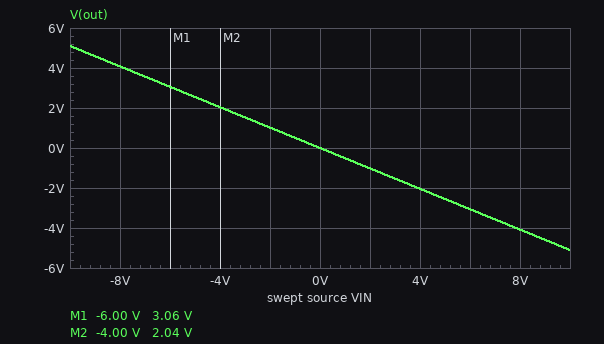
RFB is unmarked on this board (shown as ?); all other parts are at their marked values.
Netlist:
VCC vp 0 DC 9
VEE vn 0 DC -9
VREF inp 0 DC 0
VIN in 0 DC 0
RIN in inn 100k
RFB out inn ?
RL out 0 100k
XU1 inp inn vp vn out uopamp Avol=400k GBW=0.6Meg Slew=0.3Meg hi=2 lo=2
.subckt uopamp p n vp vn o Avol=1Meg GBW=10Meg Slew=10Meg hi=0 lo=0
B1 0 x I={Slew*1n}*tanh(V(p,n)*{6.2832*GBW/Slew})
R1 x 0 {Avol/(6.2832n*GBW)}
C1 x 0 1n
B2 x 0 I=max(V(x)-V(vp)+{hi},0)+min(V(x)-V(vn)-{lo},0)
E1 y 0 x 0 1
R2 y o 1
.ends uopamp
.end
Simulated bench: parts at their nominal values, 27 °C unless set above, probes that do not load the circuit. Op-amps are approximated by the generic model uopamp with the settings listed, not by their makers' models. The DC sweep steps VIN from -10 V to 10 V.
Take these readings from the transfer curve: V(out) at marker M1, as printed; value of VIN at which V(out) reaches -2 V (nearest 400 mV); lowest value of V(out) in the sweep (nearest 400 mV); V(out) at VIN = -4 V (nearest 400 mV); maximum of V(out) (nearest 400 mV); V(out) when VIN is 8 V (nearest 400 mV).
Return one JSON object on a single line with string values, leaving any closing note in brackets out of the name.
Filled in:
{"V(out) at marker M1, as printed": "3.06 V", "value of VIN at which V(out) reaches -2 V": "4.0 V", "lowest value of V(out) in the sweep": "-5.2 V", "V(out) at VIN = -4 V": "2.0 V", "maximum of V(out)": "5.2 V", "V(out) when VIN is 8 V": "-4.0 V"}
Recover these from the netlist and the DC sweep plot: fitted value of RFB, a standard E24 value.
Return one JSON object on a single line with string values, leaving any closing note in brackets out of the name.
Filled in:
{"fitted value of RFB, a standard E24 value": "51 kΩ"}
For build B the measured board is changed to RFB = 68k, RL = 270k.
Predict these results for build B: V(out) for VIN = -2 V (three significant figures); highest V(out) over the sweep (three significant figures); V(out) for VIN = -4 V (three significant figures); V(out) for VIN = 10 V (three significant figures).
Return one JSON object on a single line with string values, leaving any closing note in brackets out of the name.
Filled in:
{"V(out) for VIN = -2 V": "1.36 V", "highest V(out) over the sweep": "6.80 V", "V(out) for VIN = -4 V": "2.72 V", "V(out) for VIN = 10 V": "-6.80 V"}
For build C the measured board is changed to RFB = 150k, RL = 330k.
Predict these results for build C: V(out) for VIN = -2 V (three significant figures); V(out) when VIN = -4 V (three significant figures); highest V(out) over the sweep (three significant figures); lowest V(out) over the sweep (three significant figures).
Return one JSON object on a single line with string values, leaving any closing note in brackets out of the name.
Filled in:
{"V(out) for VIN = -2 V": "3.00 V", "V(out) when VIN = -4 V": "6.00 V", "highest V(out) over the sweep": "7.00 V", "lowest V(out) over the sweep": "-7.00 V"}
